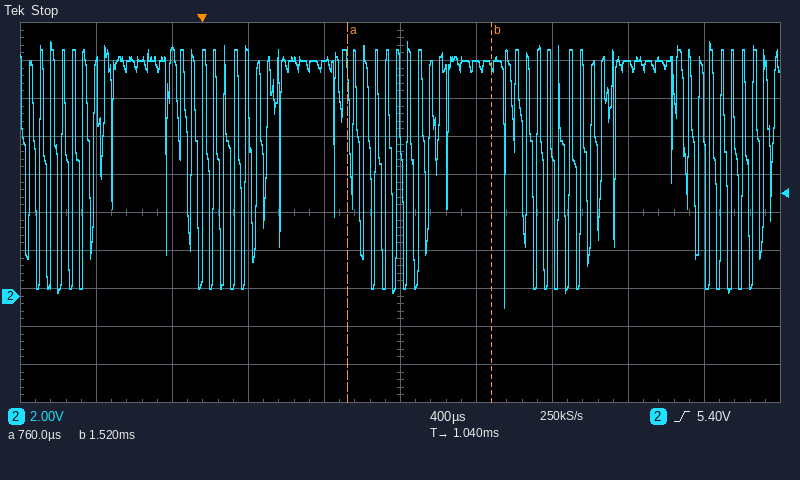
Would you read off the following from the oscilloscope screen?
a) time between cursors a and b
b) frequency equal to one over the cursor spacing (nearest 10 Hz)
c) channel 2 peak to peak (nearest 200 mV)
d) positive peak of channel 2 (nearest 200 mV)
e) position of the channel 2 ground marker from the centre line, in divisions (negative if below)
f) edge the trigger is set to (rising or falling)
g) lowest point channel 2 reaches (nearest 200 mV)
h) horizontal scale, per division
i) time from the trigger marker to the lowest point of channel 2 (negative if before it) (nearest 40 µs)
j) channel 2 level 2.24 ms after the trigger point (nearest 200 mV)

760 µs
1.32 kHz
14.0 V
13.4 V
-2.2 div
rising
-600 mV
400 µs
+1.60 ms
12.2 V
